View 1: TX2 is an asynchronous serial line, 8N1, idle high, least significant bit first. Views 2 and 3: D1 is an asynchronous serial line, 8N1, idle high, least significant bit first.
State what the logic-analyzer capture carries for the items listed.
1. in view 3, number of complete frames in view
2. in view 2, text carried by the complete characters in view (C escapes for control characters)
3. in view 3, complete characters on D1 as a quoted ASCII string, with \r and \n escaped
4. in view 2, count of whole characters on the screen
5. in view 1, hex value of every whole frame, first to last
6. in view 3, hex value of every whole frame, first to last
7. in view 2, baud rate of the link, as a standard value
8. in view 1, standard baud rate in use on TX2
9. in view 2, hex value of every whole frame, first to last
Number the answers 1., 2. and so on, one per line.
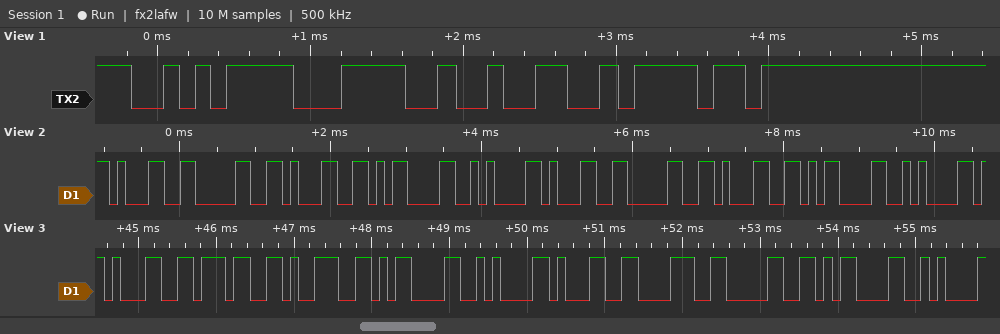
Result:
1. 10
2. "101\r\n101\r\n"
3. "179\r\n180\r\n"
4. 10
5. EA 3C 32 6F
6. 31 37 39 0D 0A 31 38 30 0D 0A
7. 9600 baud
8. 9600 baud
9. 31 30 31 0D 0A 31 30 31 0D 0A
